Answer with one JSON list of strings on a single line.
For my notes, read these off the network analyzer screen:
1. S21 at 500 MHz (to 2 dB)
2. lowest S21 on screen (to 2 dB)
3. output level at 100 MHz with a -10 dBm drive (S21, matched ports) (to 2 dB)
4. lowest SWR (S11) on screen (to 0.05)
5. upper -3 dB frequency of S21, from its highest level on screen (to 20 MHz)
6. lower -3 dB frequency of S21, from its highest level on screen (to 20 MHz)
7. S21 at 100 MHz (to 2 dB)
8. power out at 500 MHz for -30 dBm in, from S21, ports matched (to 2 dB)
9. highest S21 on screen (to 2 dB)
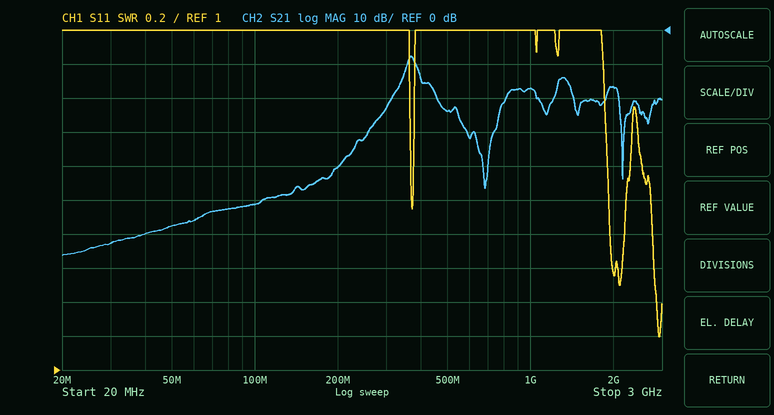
["-24 dB", "-66 dB", "-62 dBm", "1.20", "380 MHz", "360 MHz", "-52 dB", "-54 dBm", "-8 dB"]
